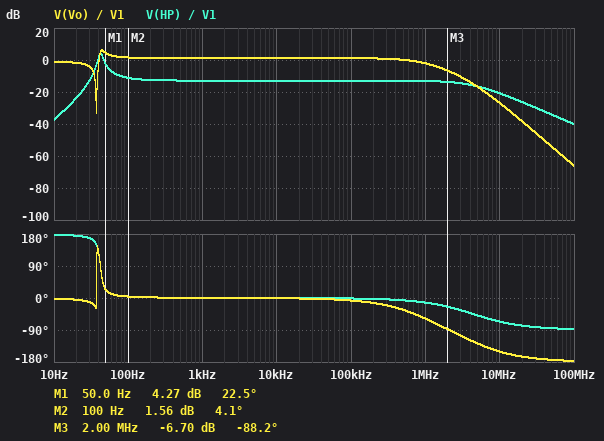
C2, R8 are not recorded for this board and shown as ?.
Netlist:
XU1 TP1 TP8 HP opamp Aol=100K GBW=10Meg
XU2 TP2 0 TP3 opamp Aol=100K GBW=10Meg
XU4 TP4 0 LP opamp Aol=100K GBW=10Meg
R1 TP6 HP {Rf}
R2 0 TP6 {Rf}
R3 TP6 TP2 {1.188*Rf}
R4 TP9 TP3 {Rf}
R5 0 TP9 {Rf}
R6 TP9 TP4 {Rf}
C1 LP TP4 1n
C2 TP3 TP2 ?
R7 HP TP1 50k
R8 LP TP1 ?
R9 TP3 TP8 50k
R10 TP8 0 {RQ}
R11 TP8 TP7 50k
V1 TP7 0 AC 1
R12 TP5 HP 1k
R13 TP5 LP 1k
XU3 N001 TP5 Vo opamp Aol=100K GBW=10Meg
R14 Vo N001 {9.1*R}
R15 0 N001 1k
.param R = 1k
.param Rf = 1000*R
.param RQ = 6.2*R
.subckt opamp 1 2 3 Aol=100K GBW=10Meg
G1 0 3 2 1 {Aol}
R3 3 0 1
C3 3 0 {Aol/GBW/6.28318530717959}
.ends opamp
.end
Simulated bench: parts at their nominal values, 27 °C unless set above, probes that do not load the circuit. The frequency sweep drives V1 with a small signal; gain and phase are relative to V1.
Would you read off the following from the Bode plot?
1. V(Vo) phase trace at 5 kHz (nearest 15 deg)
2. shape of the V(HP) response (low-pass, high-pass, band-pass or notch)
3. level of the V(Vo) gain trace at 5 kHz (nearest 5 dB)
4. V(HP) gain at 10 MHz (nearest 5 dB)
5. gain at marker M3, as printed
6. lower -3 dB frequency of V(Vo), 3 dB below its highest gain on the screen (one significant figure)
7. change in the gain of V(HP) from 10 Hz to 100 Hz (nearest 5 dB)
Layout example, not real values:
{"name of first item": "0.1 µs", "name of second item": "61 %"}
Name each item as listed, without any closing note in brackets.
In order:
{"V(Vo) phase trace at 5 kHz": "0 deg", "shape of the V(HP) response": "band-pass", "level of the V(Vo) gain trace at 5 kHz": "0 dB", "V(HP) gain at 10 MHz": "-20 dB", "gain at marker M3, as printed": "-6.70 dB", "lower -3 dB frequency of V(Vo), 3 dB below its highest gain on the screen": "40 Hz", "change in the gain of V(HP) from 10 Hz to 100 Hz": "25 dB"}
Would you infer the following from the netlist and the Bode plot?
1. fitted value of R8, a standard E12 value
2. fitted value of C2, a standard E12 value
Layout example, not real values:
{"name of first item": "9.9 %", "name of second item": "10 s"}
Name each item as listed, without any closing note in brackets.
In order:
{"fitted value of R8, a standard E12 value": "39 kΩ", "fitted value of C2, a standard E12 value": "1.8 nF"}
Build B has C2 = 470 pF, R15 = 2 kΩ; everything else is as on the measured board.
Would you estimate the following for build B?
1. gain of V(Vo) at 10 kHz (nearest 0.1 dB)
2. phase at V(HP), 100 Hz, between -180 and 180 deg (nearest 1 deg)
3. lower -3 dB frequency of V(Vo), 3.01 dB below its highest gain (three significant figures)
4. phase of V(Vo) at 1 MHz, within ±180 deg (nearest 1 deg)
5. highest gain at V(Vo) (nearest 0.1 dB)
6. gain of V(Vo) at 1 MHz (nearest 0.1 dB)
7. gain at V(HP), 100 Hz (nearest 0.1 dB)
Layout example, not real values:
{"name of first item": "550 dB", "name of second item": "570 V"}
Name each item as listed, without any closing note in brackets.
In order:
{"gain of V(Vo) at 10 kHz": "-4.0 dB", "phase at V(HP), 100 Hz, between -180 and 180 deg": "36 deg", "lower -3 dB frequency of V(Vo), 3.01 dB below its highest gain": "83.3 Hz", "phase of V(Vo) at 1 MHz, within ±180 deg": "-42 deg", "highest gain at V(Vo)": "-2.4 dB", "gain of V(Vo) at 1 MHz": "-5.4 dB", "gain at V(HP), 100 Hz": "-4.7 dB"}
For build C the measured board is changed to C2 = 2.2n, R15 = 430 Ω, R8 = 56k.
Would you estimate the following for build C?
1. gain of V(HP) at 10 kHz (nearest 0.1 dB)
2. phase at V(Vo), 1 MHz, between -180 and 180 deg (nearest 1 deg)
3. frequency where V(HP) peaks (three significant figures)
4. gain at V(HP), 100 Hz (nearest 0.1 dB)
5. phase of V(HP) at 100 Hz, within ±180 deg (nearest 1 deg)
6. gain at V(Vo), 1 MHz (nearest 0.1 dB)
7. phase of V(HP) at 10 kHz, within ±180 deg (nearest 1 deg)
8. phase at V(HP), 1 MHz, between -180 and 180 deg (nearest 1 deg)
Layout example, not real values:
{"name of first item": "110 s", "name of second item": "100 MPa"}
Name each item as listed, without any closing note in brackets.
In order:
{"gain of V(HP) at 10 kHz": "-14.5 dB", "phase at V(Vo), 1 MHz, between -180 and 180 deg": "-76 deg", "frequency where V(HP) peaks": "32.0 Hz", "gain at V(HP), 100 Hz": "-13.6 dB", "phase of V(HP) at 100 Hz, within ±180 deg": "3 deg", "gain at V(Vo), 1 MHz": "-1.5 dB", "phase of V(HP) at 10 kHz, within ±180 deg": "0 deg", "phase at V(HP), 1 MHz, between -180 and 180 deg": "-11 deg"}
